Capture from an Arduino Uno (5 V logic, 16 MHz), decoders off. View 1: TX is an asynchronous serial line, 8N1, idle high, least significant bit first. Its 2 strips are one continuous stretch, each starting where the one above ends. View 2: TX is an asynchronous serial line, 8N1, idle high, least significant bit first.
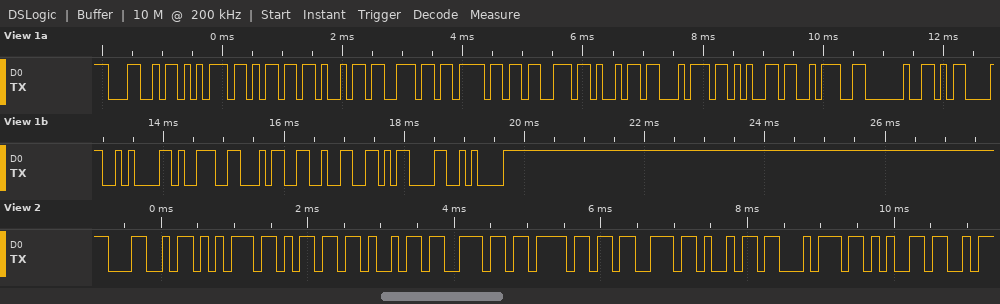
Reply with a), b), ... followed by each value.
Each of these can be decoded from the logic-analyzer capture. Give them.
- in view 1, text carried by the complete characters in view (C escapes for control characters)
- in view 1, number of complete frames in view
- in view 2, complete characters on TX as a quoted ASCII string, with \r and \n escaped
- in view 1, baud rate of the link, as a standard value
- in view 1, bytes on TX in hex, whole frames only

a) "Luminosite: \r\n942\r\n"
b) 19
c) "Luminosite"
d) 9600 baud
e) 4C 75 6D 69 6E 6F 73 69 74 65 3A 20 0D 0A 39 34 32 0D 0A
